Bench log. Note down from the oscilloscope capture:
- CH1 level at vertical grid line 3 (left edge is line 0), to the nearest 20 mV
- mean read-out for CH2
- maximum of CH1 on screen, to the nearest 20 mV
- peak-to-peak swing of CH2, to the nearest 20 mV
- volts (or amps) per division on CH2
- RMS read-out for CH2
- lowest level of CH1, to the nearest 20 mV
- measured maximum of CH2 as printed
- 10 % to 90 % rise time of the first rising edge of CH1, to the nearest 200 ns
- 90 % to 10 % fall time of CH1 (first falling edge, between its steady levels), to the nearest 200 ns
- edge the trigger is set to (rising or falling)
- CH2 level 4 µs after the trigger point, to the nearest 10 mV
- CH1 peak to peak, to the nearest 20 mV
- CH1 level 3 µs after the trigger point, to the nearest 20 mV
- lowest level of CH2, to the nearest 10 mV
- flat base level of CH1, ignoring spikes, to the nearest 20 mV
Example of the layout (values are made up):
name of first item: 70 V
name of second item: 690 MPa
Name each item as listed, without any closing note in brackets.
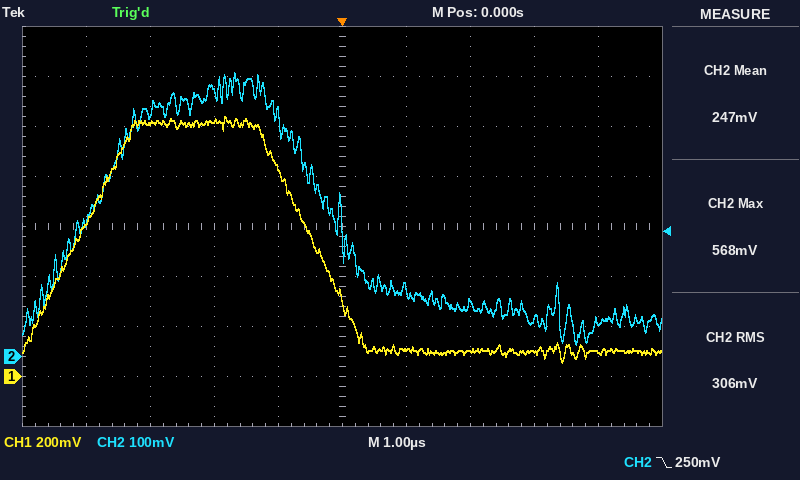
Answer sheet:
CH1 level at vertical grid line 3 (left edge is line 0), to the nearest 20 mV: 1.02 V
mean read-out for CH2: 247 mV
maximum of CH1 on screen, to the nearest 20 mV: 1.04 V
peak-to-peak swing of CH2, to the nearest 20 mV: 540 mV
volts (or amps) per division on CH2: 100 mV
RMS read-out for CH2: 306 mV
lowest level of CH1, to the nearest 20 mV: 60 mV
measured maximum of CH2 as printed: 568 mV
10 % to 90 % rise time of the first rising edge of CH1, to the nearest 200 ns: 1.4 µs
90 % to 10 % fall time of CH1 (first falling edge, between its steady levels), to the nearest 200 ns: 1.4 µs
edge the trigger is set to: falling
CH2 level 4 µs after the trigger point, to the nearest 10 mV: 70 mV
CH1 peak to peak, to the nearest 20 mV: 980 mV
CH1 level 3 µs after the trigger point, to the nearest 20 mV: 100 mV
lowest level of CH2, to the nearest 10 mV: 20 mV
flat base level of CH1, ignoring spikes, to the nearest 20 mV: 100 mV
